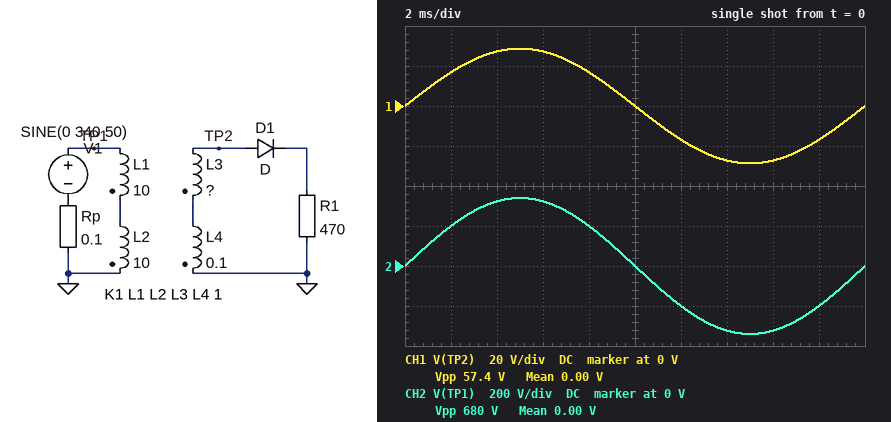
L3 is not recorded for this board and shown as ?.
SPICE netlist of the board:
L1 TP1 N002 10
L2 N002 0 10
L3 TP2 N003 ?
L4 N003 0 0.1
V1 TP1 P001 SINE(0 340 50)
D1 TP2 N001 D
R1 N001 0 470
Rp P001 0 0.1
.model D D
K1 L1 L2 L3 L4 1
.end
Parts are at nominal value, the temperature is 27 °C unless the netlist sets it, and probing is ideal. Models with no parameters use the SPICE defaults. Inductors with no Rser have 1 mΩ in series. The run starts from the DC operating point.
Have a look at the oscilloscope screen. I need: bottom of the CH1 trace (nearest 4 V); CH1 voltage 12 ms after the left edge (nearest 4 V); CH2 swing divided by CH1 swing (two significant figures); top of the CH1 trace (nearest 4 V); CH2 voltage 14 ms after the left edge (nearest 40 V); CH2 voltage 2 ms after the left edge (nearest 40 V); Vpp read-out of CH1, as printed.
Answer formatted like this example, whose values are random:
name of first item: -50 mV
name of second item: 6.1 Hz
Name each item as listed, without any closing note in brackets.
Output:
bottom of the CH1 trace: -28 V
CH1 voltage 12 ms after the left edge: -16 V
CH2 swing divided by CH1 swing: 12
top of the CH1 trace: 28 V
CH2 voltage 14 ms after the left edge: -320 V
CH2 voltage 2 ms after the left edge: 200 V
Vpp read-out of CH1, as printed: 57.4 V
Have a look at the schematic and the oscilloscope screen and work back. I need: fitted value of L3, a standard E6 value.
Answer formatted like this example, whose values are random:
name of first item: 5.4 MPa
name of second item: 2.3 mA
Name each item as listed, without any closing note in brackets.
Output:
fitted value of L3, a standard E6 value: 47 mH
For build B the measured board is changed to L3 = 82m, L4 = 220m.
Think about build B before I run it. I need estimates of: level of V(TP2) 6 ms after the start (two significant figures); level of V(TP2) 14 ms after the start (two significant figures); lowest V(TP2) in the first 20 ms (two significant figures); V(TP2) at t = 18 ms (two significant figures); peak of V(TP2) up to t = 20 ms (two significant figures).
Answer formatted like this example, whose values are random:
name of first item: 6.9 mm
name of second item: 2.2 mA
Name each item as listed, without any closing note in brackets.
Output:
level of V(TP2) 6 ms after the start: 39 V
level of V(TP2) 14 ms after the start: -39 V
lowest V(TP2) in the first 20 ms: -41 V
V(TP2) at t = 18 ms: -24 V
peak of V(TP2) up to t = 20 ms: 41 V
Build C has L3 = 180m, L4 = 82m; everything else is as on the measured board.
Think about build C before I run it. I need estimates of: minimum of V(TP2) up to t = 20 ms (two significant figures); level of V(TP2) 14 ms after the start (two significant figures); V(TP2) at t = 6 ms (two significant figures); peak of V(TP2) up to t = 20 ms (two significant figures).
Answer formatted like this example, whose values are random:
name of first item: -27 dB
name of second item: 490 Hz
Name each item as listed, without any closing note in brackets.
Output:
minimum of V(TP2) up to t = 20 ms: -38 V
level of V(TP2) 14 ms after the start: -36 V
V(TP2) at t = 6 ms: 36 V
peak of V(TP2) up to t = 20 ms: 38 V
